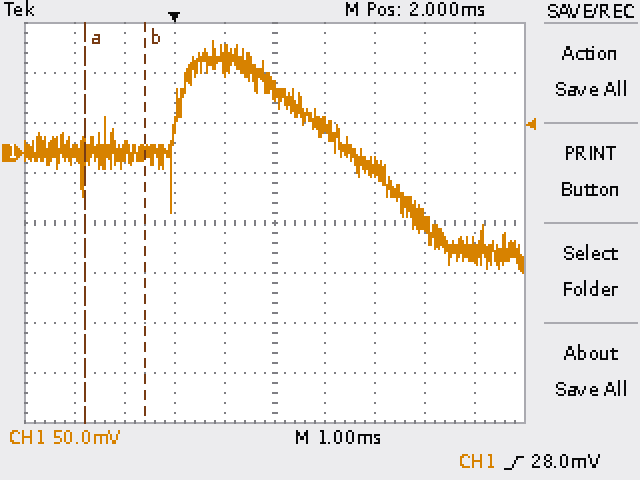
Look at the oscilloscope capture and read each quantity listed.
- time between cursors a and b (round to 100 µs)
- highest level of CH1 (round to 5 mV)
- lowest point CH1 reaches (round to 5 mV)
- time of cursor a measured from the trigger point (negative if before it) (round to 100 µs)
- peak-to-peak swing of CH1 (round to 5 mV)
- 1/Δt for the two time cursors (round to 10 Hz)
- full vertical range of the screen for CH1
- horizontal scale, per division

1.2 ms
110 mV
-120 mV
-1.8 ms
230 mV
830 Hz
400 mV
1 ms
